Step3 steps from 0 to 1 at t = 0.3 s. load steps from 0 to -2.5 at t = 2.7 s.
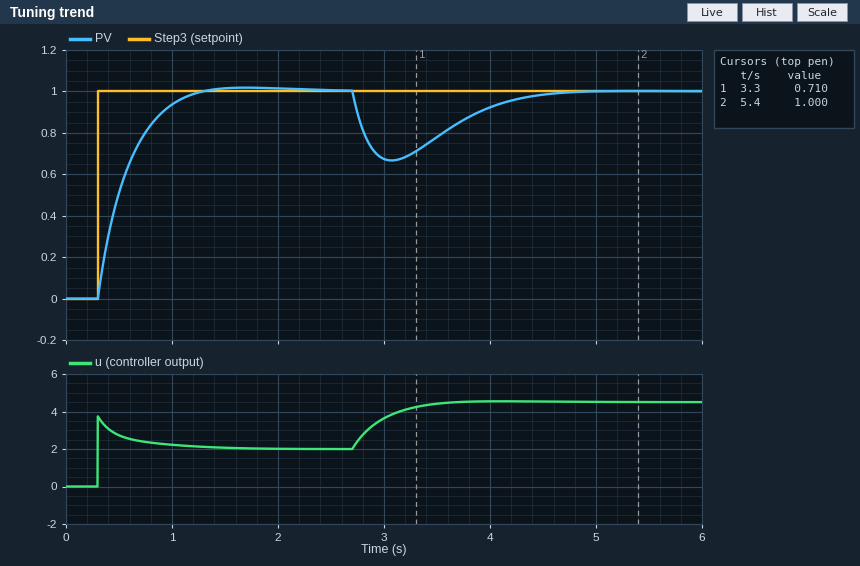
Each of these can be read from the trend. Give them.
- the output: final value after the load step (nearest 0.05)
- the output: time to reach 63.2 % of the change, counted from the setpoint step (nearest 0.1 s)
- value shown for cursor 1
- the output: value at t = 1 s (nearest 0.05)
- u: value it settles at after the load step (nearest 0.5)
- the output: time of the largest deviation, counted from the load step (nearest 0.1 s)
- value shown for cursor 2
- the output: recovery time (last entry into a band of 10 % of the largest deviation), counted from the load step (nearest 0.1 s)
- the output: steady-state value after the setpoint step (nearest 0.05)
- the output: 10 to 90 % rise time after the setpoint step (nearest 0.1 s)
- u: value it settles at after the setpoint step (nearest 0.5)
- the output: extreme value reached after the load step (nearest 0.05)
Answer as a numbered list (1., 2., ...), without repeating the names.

1. 1.00
2. 0.3 s
3. 0.710
4. 0.95
5. 4.5
6. 0.4 s
7. 1.000
8. 1.6 s
9. 1.00
10. 0.6 s
11. 2.0
12. 0.65
